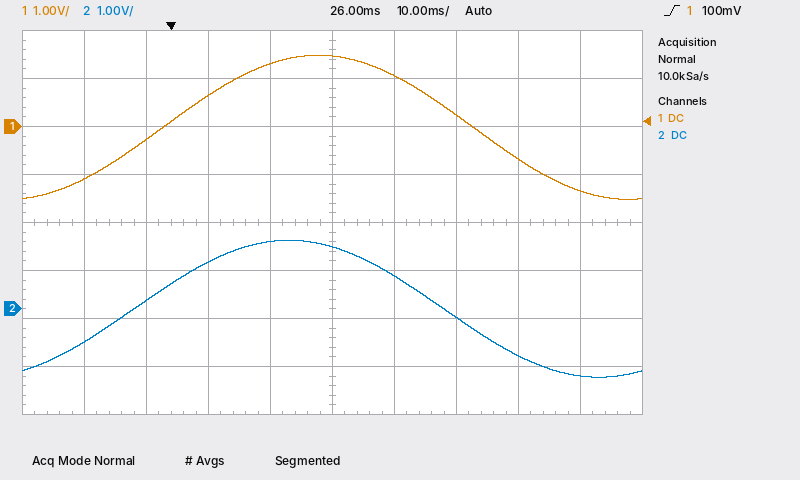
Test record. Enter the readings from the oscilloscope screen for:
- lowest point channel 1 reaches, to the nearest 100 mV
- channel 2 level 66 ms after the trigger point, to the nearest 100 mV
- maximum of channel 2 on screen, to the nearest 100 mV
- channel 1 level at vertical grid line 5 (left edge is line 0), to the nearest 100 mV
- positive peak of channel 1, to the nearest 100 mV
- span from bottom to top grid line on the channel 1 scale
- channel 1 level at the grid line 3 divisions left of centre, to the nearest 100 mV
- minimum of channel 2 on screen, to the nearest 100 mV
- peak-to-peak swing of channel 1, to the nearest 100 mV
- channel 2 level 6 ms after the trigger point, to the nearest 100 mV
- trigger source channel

-1.5 V
-1.4 V
1.4 V
1.5 V
1.5 V
8 V
-300 mV
-1.4 V
3.0 V
1.0 V
channel 1
